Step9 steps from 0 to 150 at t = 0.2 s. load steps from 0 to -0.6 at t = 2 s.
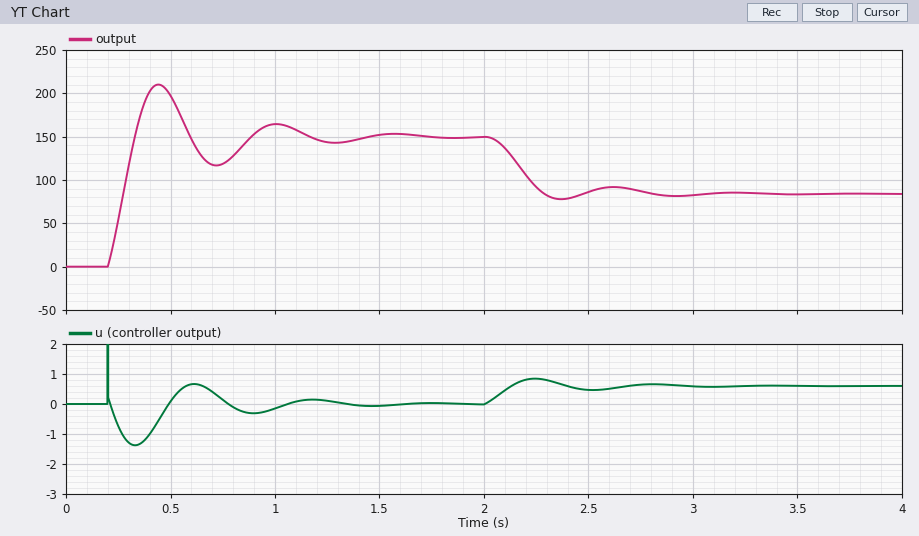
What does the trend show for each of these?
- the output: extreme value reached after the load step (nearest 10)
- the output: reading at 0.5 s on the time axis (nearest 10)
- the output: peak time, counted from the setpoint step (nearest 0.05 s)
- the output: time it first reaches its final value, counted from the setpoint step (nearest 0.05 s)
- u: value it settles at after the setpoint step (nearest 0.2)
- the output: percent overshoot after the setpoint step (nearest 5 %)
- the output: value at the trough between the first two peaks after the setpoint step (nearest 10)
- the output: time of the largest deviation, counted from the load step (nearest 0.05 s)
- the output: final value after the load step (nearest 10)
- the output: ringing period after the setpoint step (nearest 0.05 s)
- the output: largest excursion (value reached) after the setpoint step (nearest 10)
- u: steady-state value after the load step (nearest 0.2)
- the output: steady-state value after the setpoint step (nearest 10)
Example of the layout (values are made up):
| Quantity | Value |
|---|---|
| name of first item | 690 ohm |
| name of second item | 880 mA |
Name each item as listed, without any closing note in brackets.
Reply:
| Quantity | Value |
|---|---|
| the output: extreme value reached after the load step | 80 |
| the output: reading at 0.5 s on the time axis | 200 |
| the output: peak time, counted from the setpoint step | 0.25 s |
| the output: time it first reaches its final value, counted from the setpoint step | 0.15 s |
| u: value it settles at after the setpoint step | 0.0 |
| the output: percent overshoot after the setpoint step | 40 % |
| the output: value at the trough between the first two peaks after the setpoint step | 120 |
| the output: time of the largest deviation, counted from the load step | 0.35 s |
| the output: final value after the load step | 80 |
| the output: ringing period after the setpoint step | 0.55 s |
| the output: largest excursion (value reached) after the setpoint step | 210 |
| u: steady-state value after the load step | 0.6 |
| the output: steady-state value after the setpoint step | 150 |
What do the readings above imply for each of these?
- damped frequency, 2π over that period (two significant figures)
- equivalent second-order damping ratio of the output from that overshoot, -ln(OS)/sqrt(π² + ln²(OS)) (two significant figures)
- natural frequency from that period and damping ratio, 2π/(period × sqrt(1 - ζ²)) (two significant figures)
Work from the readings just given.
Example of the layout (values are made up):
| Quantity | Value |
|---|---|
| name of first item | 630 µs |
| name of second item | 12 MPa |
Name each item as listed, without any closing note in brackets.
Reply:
| Quantity | Value |
|---|---|
| damped frequency, 2π over that period | 11 rad/s |
| equivalent second-order damping ratio of the output from that overshoot, -ln(OS)/sqrt(π² + ln²(OS)) | 0.28 |
| natural frequency from that period and damping ratio, 2π/(period × sqrt(1 - ζ²)) | 12 rad/s |
